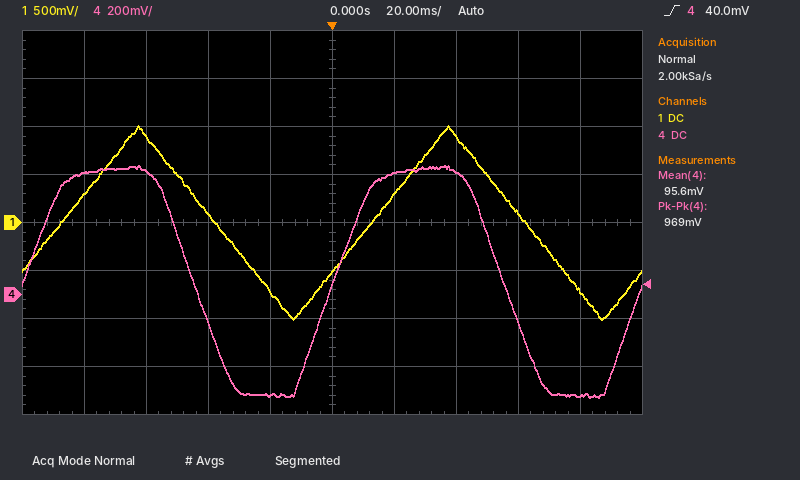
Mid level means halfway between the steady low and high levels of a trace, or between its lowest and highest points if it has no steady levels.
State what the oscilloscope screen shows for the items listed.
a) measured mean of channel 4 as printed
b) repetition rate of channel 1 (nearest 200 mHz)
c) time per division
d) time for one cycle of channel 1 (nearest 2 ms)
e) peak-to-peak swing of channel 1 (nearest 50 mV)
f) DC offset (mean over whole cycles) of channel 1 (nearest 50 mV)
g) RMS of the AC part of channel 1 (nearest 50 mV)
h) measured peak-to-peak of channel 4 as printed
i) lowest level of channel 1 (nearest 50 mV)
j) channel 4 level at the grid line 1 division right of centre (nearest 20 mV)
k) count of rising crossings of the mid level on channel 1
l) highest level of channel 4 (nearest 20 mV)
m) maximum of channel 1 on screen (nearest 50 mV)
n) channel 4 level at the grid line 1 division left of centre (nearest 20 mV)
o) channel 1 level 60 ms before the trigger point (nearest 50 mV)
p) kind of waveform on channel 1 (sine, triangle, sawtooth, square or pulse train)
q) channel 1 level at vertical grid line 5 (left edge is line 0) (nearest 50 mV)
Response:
95.6 mV
10.0 Hz
20 ms
100 ms
2.00 V
0 mV
600 mV
969 mV
-1.00 V
500 mV
2
540 mV
1.00 V
-420 mV
900 mV
triangle
-500 mV
